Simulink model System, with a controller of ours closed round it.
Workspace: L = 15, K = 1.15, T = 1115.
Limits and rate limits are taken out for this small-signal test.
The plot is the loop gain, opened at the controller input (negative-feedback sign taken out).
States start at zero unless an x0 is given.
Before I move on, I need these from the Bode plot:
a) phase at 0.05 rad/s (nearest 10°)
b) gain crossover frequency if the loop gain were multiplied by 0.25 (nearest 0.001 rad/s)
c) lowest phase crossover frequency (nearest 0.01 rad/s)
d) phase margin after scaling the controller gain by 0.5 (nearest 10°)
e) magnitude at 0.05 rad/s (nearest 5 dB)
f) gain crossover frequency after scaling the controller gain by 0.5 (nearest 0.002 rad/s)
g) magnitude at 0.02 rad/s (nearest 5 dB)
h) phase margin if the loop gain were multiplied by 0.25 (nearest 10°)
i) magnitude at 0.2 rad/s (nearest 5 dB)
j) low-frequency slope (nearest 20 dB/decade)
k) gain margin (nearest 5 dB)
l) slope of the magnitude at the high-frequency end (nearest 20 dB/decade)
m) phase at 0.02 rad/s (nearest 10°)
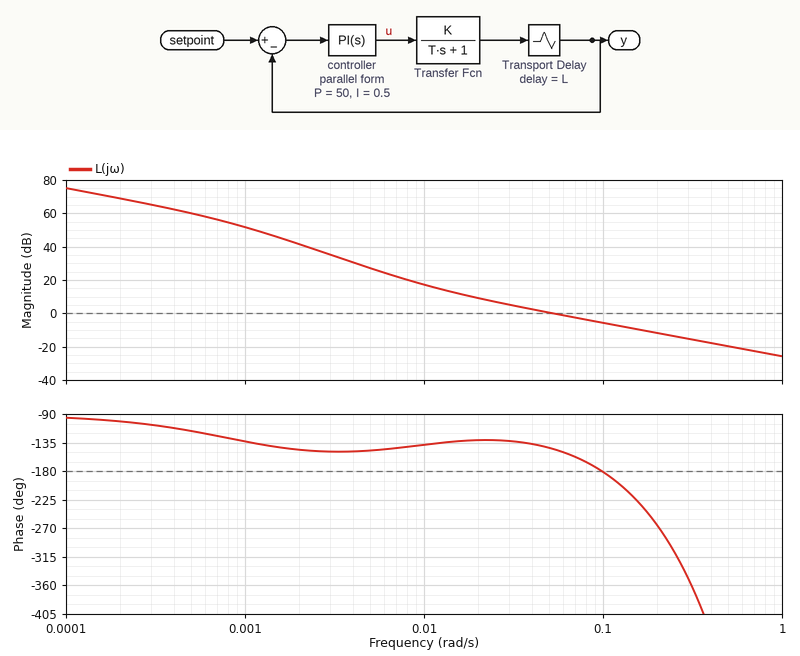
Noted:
-140°
0.015 rad/s
0.10 rad/s
50°
0 dB
0.028 rad/s
10 dB
50°
-10 dB
-20 dB/decade
5 dB
-20 dB/decade
-130°
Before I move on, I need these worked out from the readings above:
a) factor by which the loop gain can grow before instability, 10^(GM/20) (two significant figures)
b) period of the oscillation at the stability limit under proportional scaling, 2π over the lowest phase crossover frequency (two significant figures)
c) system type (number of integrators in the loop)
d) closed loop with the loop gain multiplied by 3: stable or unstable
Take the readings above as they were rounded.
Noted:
1.8
63 s
1
unstable
